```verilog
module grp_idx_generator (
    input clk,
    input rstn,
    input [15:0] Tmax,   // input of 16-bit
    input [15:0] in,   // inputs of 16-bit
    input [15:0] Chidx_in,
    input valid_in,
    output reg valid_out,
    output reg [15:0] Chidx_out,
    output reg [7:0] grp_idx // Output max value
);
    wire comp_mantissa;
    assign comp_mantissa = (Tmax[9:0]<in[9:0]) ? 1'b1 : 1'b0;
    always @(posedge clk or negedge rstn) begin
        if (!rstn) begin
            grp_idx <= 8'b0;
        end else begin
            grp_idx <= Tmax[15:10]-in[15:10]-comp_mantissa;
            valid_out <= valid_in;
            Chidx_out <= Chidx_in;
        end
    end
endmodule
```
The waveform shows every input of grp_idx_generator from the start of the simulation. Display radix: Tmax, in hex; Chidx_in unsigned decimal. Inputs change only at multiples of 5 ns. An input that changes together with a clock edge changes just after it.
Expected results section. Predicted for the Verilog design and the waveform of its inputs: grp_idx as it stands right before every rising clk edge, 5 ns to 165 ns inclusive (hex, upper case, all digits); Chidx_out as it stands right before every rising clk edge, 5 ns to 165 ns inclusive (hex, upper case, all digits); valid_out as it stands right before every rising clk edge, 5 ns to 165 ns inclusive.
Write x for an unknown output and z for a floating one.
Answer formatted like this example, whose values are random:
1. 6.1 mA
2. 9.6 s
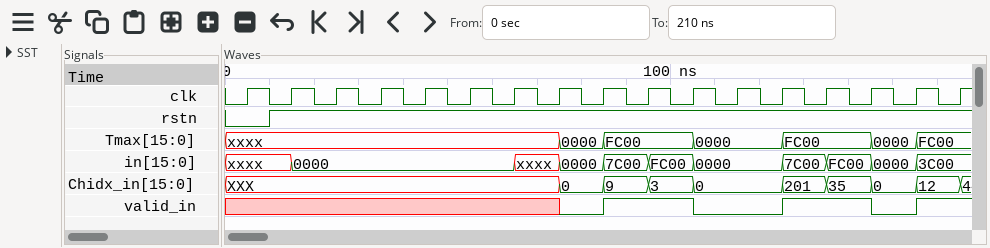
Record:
1. 00, 00, x, x, x, x, x, x, x, 00, 20, 00, 00, 00, 20, 00, 00
2. x, x, x, x, x, x, x, x, x, 0000, 0009, 0003, 0000, 0000, 00C9, 0023, 0000
3. x x x x x x x x x 0 1 1 0 0 1 1 0
